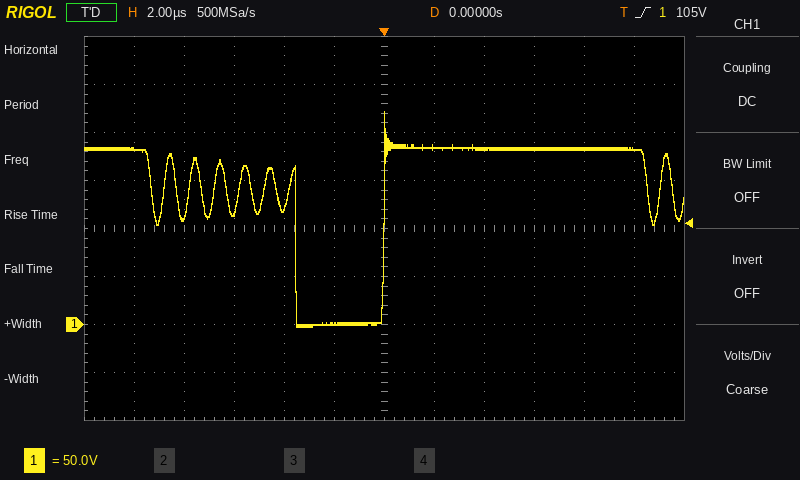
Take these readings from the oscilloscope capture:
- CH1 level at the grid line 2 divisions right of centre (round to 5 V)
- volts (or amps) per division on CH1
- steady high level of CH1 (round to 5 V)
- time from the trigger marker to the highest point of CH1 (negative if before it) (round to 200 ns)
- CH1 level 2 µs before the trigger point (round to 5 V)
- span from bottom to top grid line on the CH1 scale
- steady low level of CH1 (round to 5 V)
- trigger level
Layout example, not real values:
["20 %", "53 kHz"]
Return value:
["185 V", "50 V", "185 V", "0.0 µs", "0 V", "400 V", "0 V", "105 V"]
